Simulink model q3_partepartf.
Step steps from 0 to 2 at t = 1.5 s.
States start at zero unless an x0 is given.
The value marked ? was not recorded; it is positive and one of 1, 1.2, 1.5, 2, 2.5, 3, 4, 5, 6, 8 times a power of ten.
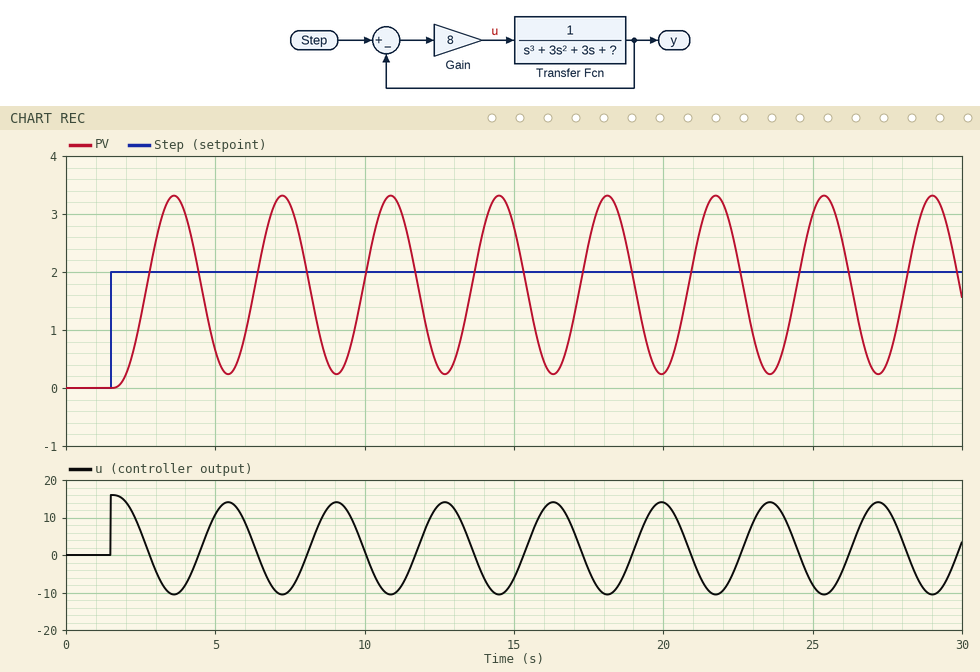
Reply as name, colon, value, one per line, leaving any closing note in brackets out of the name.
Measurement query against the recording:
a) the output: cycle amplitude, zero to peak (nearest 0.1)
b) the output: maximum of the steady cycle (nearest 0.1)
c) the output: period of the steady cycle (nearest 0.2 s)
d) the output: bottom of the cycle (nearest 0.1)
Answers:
the output: cycle amplitude, zero to peak: 1.5
the output: maximum of the steady cycle: 3.3
the output: period of the steady cycle: 3.6 s
the output: bottom of the cycle: 0.2
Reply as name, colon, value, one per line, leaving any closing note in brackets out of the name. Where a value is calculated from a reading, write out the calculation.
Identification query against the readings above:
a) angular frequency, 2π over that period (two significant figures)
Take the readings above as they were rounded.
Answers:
angular frequency, 2π over that period: 2π / 3.6 = 1.7 rad/s
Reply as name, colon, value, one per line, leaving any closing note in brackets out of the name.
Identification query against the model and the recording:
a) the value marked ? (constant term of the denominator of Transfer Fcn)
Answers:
the value marked ?: 1
